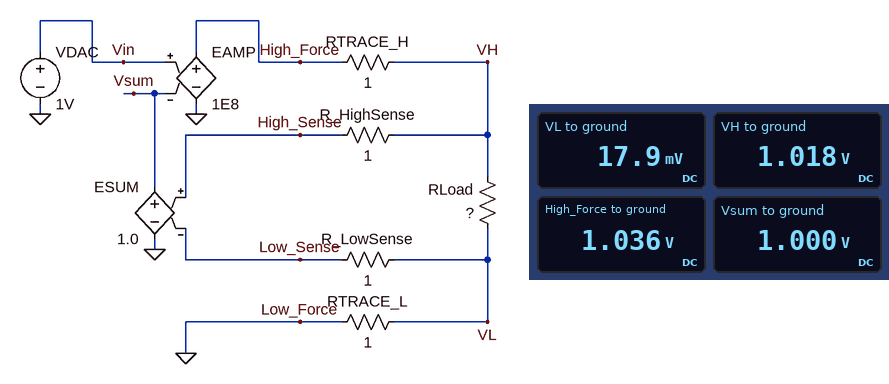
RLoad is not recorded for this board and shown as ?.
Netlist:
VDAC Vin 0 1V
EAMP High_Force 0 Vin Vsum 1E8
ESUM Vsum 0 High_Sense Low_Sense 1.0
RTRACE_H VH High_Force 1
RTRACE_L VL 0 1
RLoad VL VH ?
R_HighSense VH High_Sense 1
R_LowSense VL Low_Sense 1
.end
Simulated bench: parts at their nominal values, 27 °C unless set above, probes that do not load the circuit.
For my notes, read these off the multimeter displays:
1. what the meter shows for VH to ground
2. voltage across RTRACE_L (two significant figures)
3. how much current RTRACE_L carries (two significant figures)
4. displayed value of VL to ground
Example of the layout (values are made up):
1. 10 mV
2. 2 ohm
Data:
1. 1.018 V
2. 18 mV
3. 18 mA
4. 17.9 mV
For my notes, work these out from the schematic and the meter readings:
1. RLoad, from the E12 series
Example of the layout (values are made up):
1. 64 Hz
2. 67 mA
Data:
1. 56 Ω
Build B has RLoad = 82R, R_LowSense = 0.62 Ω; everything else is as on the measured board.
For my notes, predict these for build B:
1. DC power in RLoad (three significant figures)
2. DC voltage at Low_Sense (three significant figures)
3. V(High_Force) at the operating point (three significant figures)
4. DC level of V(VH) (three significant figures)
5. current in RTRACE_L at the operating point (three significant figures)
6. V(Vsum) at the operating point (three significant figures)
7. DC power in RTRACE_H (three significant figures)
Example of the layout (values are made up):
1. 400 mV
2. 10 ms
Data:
1. 12.2 mW
2. 12.2 mV
3. 1.02 V
4. 1.01 V
5. 12.2 mA
6. 1.00 V
7. 149 µW
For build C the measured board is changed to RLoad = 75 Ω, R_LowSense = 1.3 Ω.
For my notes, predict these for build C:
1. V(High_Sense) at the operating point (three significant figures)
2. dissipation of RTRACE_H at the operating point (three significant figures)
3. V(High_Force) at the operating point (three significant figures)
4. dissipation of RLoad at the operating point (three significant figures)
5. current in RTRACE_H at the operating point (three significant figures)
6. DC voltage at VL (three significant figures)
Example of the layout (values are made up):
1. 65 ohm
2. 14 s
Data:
1. 1.01 V
2. 178 µW
3. 1.03 V
4. 13.3 mW
5. 13.3 mA
6. 13.3 mV
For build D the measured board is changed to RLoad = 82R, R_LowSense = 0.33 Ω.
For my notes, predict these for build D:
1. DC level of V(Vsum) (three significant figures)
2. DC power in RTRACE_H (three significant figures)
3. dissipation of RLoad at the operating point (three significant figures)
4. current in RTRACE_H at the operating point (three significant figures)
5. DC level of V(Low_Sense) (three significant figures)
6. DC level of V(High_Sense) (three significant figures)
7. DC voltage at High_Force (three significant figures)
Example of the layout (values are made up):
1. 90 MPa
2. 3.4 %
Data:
1. 1.00 V
2. 149 µW
3. 12.2 mW
4. 12.2 mA
5. 12.2 mV
6. 1.01 V
7. 1.02 V
